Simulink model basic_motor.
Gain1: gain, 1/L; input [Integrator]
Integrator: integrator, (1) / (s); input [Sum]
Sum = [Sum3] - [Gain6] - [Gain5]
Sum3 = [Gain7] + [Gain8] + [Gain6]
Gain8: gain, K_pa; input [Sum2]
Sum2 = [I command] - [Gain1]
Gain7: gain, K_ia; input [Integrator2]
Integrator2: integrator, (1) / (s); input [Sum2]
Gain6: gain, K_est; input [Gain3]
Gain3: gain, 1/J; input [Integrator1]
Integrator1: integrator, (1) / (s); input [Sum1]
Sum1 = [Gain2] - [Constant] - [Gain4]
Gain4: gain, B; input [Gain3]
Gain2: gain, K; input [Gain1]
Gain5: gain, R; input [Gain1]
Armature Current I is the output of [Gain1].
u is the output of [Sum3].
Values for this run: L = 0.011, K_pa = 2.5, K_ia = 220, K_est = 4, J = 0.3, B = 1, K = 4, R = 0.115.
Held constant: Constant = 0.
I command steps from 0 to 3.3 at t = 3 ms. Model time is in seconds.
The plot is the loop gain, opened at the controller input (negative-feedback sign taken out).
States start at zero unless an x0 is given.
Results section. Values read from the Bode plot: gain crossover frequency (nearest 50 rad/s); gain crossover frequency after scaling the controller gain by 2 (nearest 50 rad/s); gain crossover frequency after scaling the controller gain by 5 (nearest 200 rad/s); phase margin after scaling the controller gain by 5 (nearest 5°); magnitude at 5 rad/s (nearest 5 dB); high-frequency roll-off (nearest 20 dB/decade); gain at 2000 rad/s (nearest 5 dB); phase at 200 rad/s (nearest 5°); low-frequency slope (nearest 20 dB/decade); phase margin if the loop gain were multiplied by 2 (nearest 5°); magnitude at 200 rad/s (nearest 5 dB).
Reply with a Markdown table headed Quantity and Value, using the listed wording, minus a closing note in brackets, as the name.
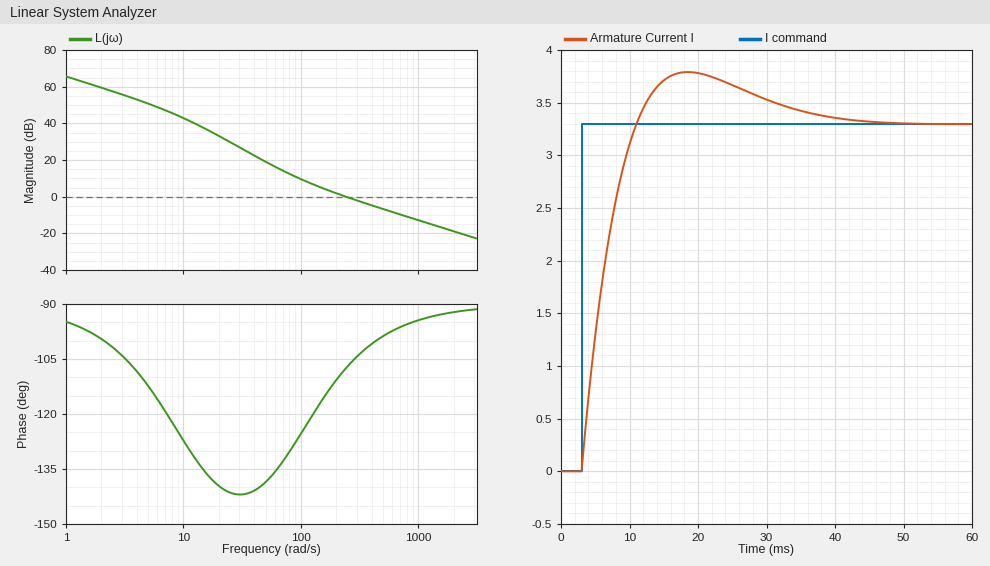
| Quantity | Value |
|---|---|
| gain crossover frequency | 250 rad/s |
| gain crossover frequency after scaling the controller gain by 2 | 450 rad/s |
| gain crossover frequency after scaling the controller gain by 5 | 1200 rad/s |
| phase margin after scaling the controller gain by 5 | 85° |
| magnitude at 5 rad/s | 50 dB |
| high-frequency roll-off | -20 dB/decade |
| gain at 2000 rad/s | -20 dB |
| phase at 200 rad/s | -110° |
| low-frequency slope | -20 dB/decade |
| phase margin if the loop gain were multiplied by 2 | 80° |
| magnitude at 200 rad/s | 0 dB |
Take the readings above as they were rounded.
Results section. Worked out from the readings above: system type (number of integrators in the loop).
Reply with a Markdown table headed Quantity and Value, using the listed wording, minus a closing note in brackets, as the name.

| Quantity | Value |
|---|---|
| system type | 1 |
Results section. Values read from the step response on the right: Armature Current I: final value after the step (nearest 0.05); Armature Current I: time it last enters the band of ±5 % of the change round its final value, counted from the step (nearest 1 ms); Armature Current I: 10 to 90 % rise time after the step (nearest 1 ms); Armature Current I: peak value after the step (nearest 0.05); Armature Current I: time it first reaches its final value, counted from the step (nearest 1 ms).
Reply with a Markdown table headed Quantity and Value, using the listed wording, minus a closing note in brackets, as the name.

| Quantity | Value |
|---|---|
| Armature Current I: final value after the step | 3.30 |
| Armature Current I: time it last enters the band of ±5 % of the change round its final value, counted from the step | 30 ms |
| Armature Current I: 10 to 90 % rise time after the step | 6 ms |
| Armature Current I: peak value after the step | 3.80 |
| Armature Current I: time it first reaches its final value, counted from the step | 8 ms |
